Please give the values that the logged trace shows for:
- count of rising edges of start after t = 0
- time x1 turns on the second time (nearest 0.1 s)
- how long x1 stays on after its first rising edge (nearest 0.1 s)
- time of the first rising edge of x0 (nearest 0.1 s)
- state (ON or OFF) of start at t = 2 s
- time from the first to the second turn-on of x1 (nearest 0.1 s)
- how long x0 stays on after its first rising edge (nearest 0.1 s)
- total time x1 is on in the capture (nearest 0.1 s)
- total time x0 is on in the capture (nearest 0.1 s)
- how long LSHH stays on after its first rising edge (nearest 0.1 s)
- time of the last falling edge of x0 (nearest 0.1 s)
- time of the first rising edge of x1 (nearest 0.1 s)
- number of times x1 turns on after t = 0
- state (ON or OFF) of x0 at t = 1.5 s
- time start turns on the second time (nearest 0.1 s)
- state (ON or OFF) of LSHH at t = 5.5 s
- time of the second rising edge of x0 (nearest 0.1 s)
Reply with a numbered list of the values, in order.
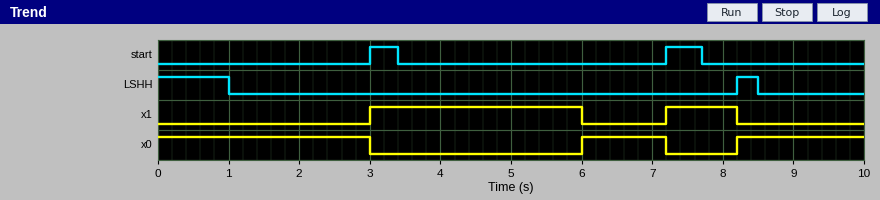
1. 2
2. 7.2 s
3. 3.0 s
4. 6.0 s
5. OFF
6. 4.2 s
7. 1.2 s
8. 4.0 s
9. 6.0 s
10. 0.3 s
11. 7.2 s
12. 3.0 s
13. 2
14. ON
15. 7.2 s
16. OFF
17. 8.2 s
